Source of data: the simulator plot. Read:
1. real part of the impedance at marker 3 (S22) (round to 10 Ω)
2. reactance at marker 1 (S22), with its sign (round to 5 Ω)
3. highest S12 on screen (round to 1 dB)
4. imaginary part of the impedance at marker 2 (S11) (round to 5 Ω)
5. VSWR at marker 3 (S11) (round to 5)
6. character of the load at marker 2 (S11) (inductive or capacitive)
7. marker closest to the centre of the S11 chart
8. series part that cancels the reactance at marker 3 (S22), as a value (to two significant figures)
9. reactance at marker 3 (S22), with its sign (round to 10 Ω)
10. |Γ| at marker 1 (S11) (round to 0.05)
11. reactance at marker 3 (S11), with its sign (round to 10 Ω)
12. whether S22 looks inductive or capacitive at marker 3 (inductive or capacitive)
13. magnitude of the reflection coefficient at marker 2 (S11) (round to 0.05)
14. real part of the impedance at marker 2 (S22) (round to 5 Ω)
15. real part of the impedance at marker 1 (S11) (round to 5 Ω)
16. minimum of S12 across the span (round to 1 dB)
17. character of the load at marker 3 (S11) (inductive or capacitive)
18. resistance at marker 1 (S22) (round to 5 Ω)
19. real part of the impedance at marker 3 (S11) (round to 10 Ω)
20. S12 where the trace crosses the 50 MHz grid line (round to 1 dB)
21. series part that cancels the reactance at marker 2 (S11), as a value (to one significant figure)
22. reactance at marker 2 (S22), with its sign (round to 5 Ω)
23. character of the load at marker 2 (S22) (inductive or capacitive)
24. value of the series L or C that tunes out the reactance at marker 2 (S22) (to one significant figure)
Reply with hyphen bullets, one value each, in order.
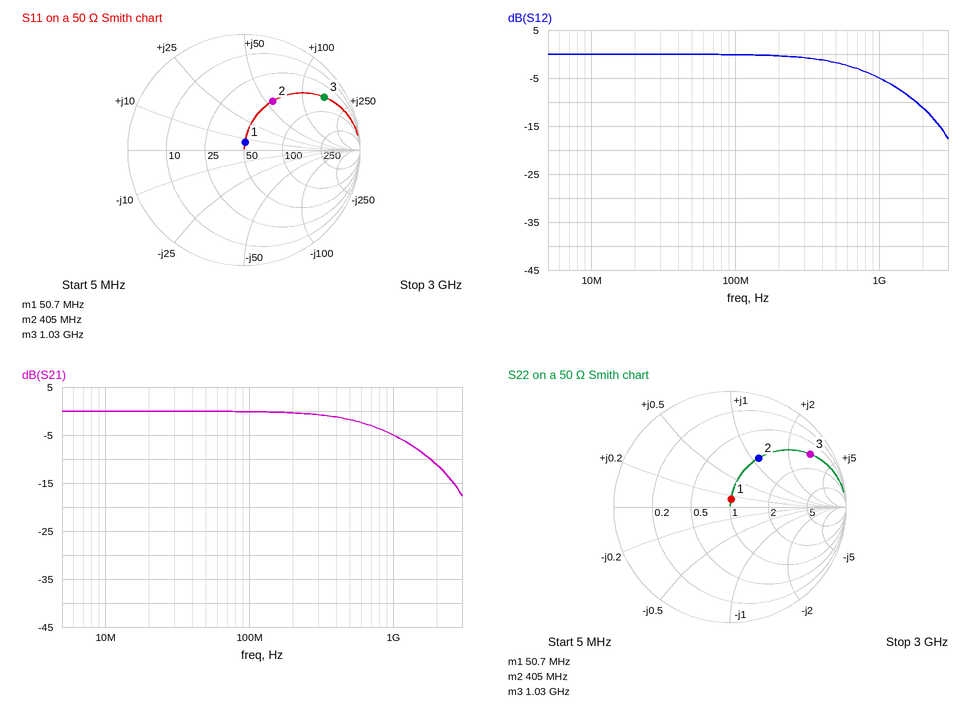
- 50 Ω
- +5 Ω
- 0 dB
- +55 Ω
- 10
- inductive
- marker 1
- 1.0 pF
- +150 Ω
- 0.05
- +150 Ω
- inductive
- 0.50
- 50 Ω
- 50 Ω
- -18 dB
- inductive
- 50 Ω
- 50 Ω
- 0 dB
- 7 pF
- +55 Ω
- inductive
- 7 pF
